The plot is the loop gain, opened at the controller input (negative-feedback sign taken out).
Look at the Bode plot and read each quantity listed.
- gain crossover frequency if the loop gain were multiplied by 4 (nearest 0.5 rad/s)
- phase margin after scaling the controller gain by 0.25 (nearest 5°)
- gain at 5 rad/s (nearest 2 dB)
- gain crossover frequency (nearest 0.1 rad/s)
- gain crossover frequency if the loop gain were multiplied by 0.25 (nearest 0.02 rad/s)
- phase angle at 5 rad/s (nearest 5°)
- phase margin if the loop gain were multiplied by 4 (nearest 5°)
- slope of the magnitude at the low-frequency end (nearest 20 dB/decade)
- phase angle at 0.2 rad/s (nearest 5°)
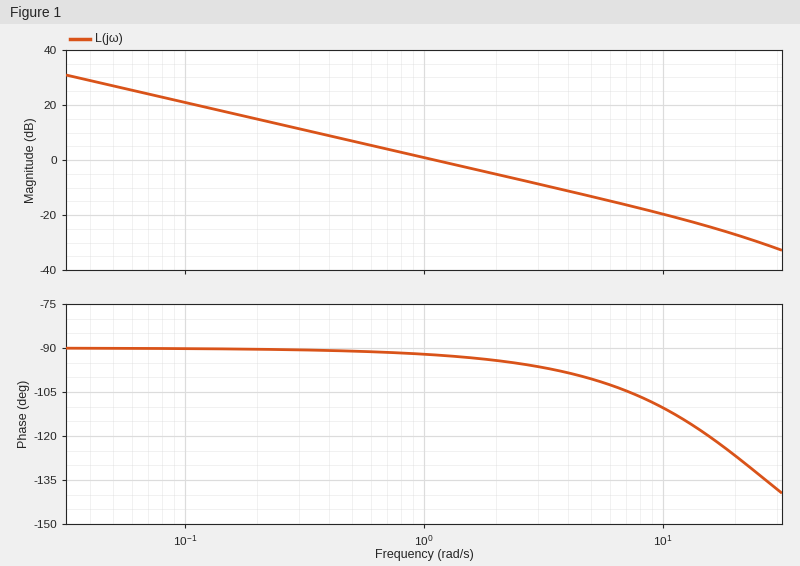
4.5 rad/s
90°
-14 dB
1.1 rad/s
0.28 rad/s
-100°
80°
-20 dB/decade
-90°
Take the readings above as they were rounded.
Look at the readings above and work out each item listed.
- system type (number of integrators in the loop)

1
